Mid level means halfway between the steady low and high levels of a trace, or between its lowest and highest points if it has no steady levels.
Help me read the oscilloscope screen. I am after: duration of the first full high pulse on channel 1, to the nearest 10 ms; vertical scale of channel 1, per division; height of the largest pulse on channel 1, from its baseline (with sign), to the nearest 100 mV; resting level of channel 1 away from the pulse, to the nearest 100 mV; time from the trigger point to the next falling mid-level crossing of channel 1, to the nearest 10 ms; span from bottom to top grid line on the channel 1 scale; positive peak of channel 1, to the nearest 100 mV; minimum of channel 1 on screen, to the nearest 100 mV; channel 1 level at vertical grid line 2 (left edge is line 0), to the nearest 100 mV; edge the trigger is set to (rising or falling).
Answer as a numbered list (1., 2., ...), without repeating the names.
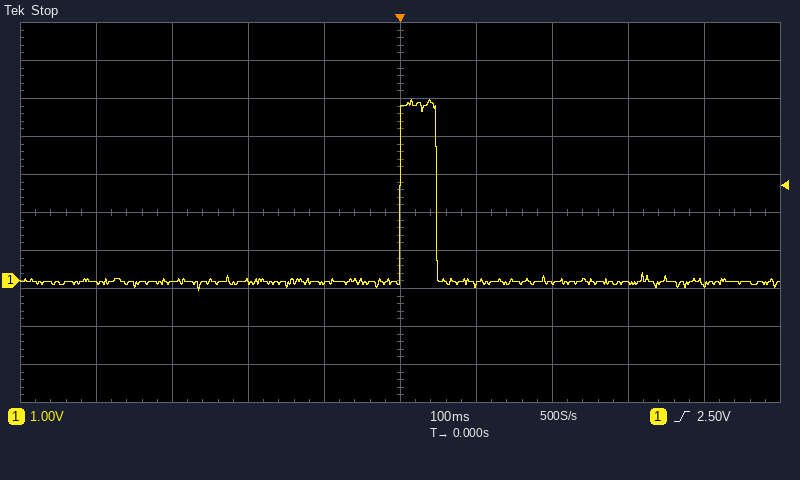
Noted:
1. 50 ms
2. 1 V
3. +4.8 V
4. 0.0 V
5. 50 ms
6. 10 V
7. 4.8 V
8. -300 mV
9. -100 mV
10. rising
